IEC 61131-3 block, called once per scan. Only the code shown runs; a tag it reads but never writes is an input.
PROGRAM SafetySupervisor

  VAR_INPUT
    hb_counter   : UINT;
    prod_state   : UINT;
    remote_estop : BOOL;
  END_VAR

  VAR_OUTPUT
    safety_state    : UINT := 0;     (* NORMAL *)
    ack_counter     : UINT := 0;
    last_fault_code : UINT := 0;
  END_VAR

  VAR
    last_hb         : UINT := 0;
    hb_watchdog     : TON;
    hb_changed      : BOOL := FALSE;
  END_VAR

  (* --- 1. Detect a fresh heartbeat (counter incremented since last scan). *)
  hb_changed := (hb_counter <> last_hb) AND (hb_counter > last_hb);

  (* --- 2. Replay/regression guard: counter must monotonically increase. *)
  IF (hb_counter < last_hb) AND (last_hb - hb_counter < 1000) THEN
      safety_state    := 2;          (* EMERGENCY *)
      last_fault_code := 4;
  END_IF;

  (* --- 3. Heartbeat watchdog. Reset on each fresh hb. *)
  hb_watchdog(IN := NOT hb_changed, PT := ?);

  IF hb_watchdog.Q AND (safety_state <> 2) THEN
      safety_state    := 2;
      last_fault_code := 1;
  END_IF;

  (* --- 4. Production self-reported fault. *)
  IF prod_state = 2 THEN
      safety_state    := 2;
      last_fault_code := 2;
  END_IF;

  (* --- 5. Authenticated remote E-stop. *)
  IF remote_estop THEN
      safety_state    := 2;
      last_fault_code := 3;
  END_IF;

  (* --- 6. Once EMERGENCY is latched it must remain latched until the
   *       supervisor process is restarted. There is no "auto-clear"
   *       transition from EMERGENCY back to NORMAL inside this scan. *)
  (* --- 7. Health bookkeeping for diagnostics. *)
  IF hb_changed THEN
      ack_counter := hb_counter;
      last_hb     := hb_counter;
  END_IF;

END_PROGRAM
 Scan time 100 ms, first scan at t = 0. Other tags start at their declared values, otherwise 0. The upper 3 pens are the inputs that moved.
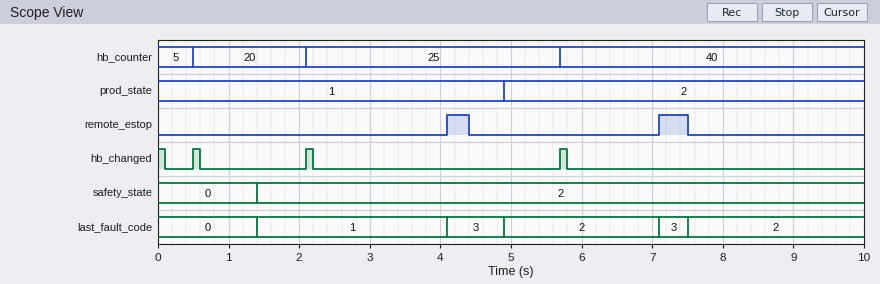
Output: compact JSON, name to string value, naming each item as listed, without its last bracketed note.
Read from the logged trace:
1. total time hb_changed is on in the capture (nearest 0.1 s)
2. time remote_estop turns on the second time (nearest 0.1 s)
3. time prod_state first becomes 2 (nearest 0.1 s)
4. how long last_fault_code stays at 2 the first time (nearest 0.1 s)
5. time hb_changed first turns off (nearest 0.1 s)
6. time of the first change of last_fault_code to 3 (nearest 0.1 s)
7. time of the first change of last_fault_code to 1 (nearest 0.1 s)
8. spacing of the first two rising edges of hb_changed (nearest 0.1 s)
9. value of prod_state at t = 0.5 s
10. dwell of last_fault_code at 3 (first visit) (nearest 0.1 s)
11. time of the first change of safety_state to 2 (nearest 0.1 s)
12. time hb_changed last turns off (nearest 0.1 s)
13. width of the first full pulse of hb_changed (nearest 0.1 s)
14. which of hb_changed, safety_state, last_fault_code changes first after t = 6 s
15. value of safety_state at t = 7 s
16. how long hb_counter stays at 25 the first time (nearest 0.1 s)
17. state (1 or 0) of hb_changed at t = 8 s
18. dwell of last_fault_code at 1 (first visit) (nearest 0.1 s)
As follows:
{"total time hb_changed is on in the capture": "0.4 s", "time remote_estop turns on the second time": "7.1 s", "time prod_state first becomes 2": "4.9 s", "how long last_fault_code stays at 2 the first time": "2.2 s", "time hb_changed first turns off": "0.1 s", "time of the first change of last_fault_code to 3": "4.1 s", "time of the first change of last_fault_code to 1": "1.4 s", "spacing of the first two rising edges of hb_changed": "1.6 s", "value of prod_state at t = 0.5 s": "1", "dwell of last_fault_code at 3 (first visit)": "0.8 s", "time of the first change of safety_state to 2": "1.4 s", "time hb_changed last turns off": "5.8 s", "width of the first full pulse of hb_changed": "0.1 s", "which of hb_changed, safety_state, last_fault_code changes first after t = 6 s": "last_fault_code", "value of safety_state at t = 7 s": "2", "how long hb_counter stays at 25 the first time": "3.6 s", "state (1 or 0) of hb_changed at t = 8 s": "0", "dwell of last_fault_code at 1 (first visit)": "2.7 s"}
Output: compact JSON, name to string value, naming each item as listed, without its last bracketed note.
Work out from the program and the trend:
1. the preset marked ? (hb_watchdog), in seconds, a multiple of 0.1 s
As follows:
{"the preset marked ? (hb_watchdog), in seconds, a multiple of 0.1 s": "0.8 s"}
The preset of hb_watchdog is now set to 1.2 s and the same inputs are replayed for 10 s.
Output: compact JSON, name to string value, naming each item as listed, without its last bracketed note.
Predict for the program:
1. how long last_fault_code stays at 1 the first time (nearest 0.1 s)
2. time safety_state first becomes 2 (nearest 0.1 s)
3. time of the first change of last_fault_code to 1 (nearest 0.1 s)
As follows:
{"how long last_fault_code stays at 1 the first time": "2.3 s", "time safety_state first becomes 2": "1.8 s", "time of the first change of last_fault_code to 1": "1.8 s"}
